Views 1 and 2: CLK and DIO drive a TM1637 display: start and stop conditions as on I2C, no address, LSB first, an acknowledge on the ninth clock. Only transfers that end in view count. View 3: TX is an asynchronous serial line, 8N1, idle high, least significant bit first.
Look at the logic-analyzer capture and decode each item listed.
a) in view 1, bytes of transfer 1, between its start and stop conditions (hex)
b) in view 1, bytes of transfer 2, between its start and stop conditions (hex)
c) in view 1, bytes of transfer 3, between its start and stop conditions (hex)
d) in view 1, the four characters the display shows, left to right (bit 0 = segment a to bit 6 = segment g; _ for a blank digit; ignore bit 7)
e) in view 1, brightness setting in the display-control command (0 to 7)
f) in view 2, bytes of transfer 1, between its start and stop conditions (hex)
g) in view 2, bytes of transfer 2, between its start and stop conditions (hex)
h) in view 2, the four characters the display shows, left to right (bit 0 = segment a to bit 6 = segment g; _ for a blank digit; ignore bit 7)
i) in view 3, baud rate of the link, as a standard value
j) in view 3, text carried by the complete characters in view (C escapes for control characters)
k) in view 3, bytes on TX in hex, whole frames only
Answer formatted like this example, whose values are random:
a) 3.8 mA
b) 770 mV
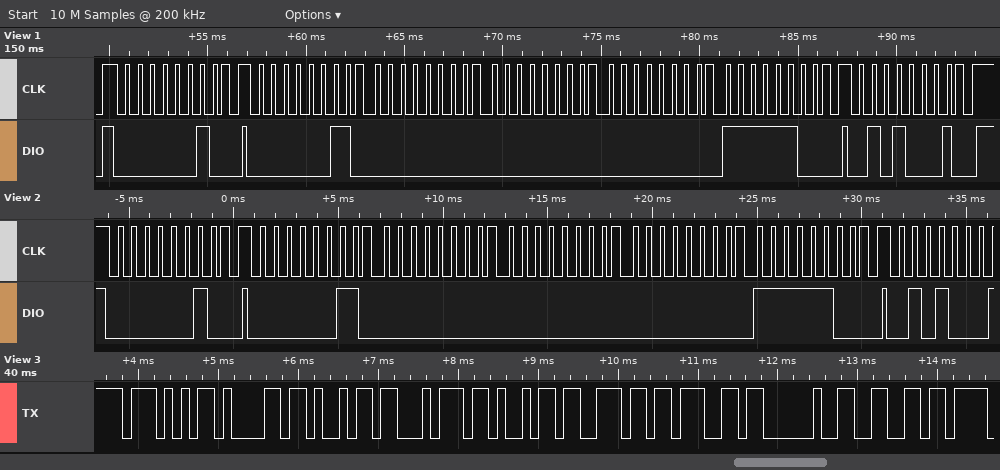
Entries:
a) 40
b) C0 00 00 00 3F
c) 8A
d) ___0
e) 2
f) 40
g) C0 00 00 00 3F
h) ___0
i) 9600 baud
j) "Waiting f"
k) 57 61 69 74 69 6E 67 20 66
